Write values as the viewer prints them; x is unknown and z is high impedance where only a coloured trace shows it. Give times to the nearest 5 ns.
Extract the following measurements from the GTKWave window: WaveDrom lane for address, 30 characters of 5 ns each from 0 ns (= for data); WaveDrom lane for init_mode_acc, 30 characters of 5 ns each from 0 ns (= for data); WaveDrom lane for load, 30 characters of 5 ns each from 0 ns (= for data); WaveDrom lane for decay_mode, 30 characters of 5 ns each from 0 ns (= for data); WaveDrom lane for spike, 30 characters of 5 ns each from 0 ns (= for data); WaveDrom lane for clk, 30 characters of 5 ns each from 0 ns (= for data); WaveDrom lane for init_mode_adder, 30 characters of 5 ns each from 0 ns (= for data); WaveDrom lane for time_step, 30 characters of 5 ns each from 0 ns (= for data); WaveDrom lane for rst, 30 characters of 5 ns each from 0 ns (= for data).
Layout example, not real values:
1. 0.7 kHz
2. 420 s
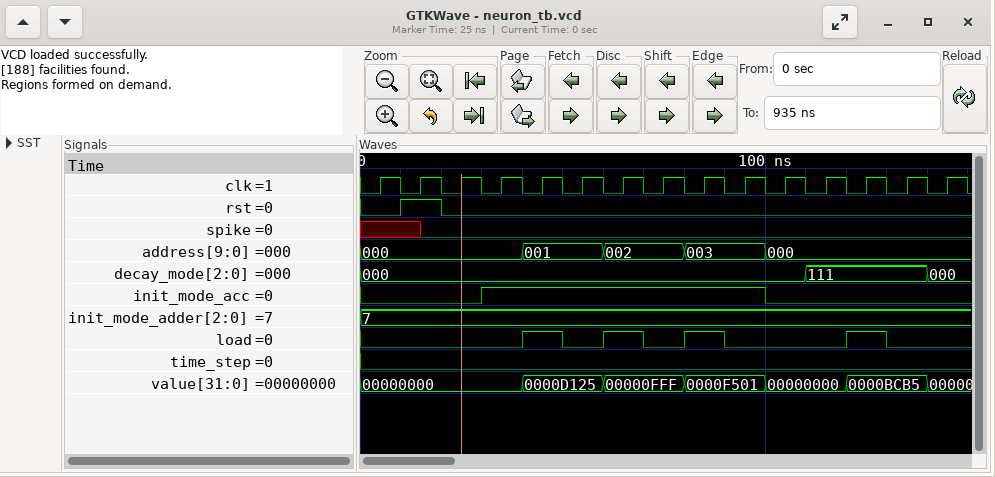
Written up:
1. {name: 'address', wave: '=.......=...=...=...=.........', data: '000 001 002 003 000'}
2. {name: 'init_mode_acc', wave: '0.....1.............0.........'}
3. {name: 'load', wave: '0.......1.0.1.0.1.0.....1.0...'}
4. {name: 'decay_mode', wave: '=.....................=.....=.', data: '000 111 000'}
5. {name: 'spike', wave: 'x..0..........................'}
6. {name: 'clk', wave: '010101010101010101010101010101'}
7. {name: 'init_mode_adder', wave: '=.............................', data: '7'}
8. {name: 'time_step', wave: '0.............................'}
9. {name: 'rst', wave: '0.1.0.........................'}
